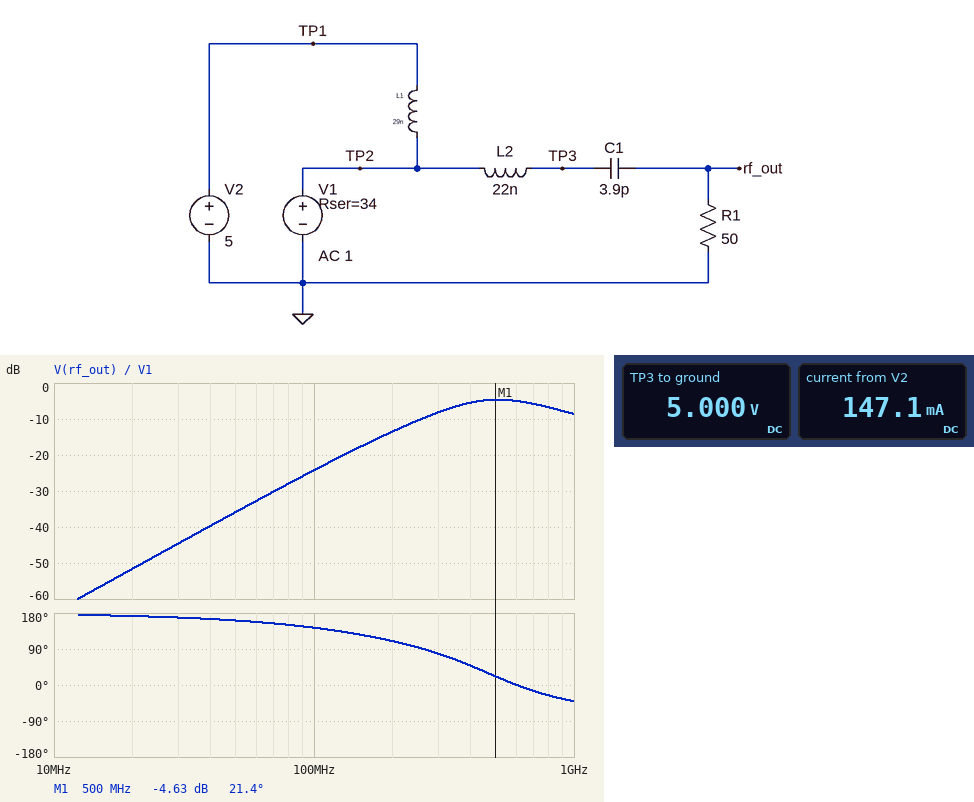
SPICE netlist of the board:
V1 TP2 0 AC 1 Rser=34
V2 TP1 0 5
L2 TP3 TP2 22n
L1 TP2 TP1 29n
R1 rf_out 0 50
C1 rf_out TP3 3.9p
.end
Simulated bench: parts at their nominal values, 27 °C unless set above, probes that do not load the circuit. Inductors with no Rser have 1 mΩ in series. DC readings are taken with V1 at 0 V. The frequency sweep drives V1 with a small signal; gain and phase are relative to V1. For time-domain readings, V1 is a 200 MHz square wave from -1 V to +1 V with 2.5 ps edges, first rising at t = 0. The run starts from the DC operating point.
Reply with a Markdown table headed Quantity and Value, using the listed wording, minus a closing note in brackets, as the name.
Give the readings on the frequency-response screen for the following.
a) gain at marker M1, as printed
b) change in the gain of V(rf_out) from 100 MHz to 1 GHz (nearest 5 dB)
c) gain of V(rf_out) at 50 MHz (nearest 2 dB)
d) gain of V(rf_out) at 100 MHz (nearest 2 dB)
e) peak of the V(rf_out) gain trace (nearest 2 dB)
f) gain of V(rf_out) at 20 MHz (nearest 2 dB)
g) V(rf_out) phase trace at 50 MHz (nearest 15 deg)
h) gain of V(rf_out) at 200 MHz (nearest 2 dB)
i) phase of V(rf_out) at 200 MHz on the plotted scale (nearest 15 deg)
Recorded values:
| Quantity | Value |
|---|---|
| gain at marker M1, as printed | -4.63 dB |
| change in the gain of V(rf_out) from 100 MHz to 1 GHz | 15 dB |
| gain of V(rf_out) at 50 MHz | -36 dB |
| gain of V(rf_out) at 100 MHz | -24 dB |
| peak of the V(rf_out) gain trace | -4 dB |
| gain of V(rf_out) at 20 MHz | -52 dB |
| V(rf_out) phase trace at 50 MHz | 165 deg |
| gain of V(rf_out) at 200 MHz | -14 dB |
| phase of V(rf_out) at 200 MHz on the plotted scale | 105 deg |
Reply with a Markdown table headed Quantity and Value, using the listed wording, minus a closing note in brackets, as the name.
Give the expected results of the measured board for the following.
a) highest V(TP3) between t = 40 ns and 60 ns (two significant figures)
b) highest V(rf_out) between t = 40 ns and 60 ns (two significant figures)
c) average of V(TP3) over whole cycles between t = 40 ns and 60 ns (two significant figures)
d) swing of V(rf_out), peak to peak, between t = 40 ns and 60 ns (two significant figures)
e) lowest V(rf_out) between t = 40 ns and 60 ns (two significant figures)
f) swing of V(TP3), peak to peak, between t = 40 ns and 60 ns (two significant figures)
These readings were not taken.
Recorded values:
| Quantity | Value |
|---|---|
| highest V(TP3) between t = 40 ns and 60 ns | 6.5 V |
| highest V(rf_out) between t = 40 ns and 60 ns | 560 mV |
| average of V(TP3) over whole cycles between t = 40 ns and 60 ns | 5.0 V |
| swing of V(rf_out), peak to peak, between t = 40 ns and 60 ns | 1.1 V |
| lowest V(rf_out) between t = 40 ns and 60 ns | -560 mV |
| swing of V(TP3), peak to peak, between t = 40 ns and 60 ns | 3.1 V |
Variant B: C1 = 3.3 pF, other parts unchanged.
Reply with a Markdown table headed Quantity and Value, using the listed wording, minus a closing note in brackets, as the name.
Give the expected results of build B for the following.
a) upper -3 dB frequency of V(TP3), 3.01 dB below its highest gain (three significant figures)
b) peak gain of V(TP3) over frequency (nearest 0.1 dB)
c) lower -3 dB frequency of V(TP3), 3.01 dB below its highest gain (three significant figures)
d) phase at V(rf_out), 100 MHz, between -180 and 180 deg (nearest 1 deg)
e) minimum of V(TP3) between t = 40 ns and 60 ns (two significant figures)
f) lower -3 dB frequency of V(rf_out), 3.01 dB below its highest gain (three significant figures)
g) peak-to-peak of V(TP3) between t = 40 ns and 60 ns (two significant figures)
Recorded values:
| Quantity | Value |
|---|---|
| upper -3 dB frequency of V(TP3), 3.01 dB below its highest gain | 710 MHz |
| peak gain of V(TP3) over frequency | 2.1 dB |
| lower -3 dB frequency of V(TP3), 3.01 dB below its highest gain | 213 MHz |
| phase at V(rf_out), 100 MHz, between -180 and 180 deg | 145 deg |
| minimum of V(TP3) between t = 40 ns and 60 ns | 3.4 V |
| lower -3 dB frequency of V(rf_out), 3.01 dB below its highest gain | 353 MHz |
| peak-to-peak of V(TP3) between t = 40 ns and 60 ns | 3.2 V |
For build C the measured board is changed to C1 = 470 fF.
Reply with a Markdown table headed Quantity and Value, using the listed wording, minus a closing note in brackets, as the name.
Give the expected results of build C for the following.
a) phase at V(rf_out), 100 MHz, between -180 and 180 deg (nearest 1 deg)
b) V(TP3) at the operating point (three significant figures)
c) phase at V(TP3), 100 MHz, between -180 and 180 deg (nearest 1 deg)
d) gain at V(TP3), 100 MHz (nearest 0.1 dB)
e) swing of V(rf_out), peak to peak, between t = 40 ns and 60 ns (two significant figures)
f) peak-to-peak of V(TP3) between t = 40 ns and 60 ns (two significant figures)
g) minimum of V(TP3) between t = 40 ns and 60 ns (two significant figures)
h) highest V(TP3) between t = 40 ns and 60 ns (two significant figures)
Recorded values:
| Quantity | Value |
|---|---|
| phase at V(rf_out), 100 MHz, between -180 and 180 deg | 151 deg |
| V(TP3) at the operating point | 5.00 V |
| phase at V(TP3), 100 MHz, between -180 and 180 deg | 62 deg |
| gain at V(TP3), 100 MHz | -6.4 dB |
| swing of V(rf_out), peak to peak, between t = 40 ns and 60 ns | 640 mV |
| peak-to-peak of V(TP3) between t = 40 ns and 60 ns | 5.1 V |
| minimum of V(TP3) between t = 40 ns and 60 ns | 2.4 V |
| highest V(TP3) between t = 40 ns and 60 ns | 7.6 V |
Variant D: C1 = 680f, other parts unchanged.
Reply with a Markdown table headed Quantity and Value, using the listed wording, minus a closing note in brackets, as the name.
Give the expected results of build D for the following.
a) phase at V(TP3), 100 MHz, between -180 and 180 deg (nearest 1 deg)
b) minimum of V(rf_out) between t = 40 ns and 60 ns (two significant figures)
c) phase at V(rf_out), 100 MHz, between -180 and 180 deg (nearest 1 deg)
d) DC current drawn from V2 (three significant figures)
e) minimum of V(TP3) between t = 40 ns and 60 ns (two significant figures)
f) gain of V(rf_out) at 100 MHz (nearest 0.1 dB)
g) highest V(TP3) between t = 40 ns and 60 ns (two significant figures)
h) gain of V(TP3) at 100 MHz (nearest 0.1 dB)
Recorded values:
| Quantity | Value |
|---|---|
| phase at V(TP3), 100 MHz, between -180 and 180 deg | 62 deg |
| minimum of V(rf_out) between t = 40 ns and 60 ns | -360 mV |
| phase at V(rf_out), 100 MHz, between -180 and 180 deg | 150 deg |
| DC current drawn from V2 | 147 mA |
| minimum of V(TP3) between t = 40 ns and 60 ns | 2.6 V |
| gain of V(rf_out) at 100 MHz | -39.8 dB |
| highest V(TP3) between t = 40 ns and 60 ns | 7.4 V |
| gain of V(TP3) at 100 MHz | -6.4 dB |
